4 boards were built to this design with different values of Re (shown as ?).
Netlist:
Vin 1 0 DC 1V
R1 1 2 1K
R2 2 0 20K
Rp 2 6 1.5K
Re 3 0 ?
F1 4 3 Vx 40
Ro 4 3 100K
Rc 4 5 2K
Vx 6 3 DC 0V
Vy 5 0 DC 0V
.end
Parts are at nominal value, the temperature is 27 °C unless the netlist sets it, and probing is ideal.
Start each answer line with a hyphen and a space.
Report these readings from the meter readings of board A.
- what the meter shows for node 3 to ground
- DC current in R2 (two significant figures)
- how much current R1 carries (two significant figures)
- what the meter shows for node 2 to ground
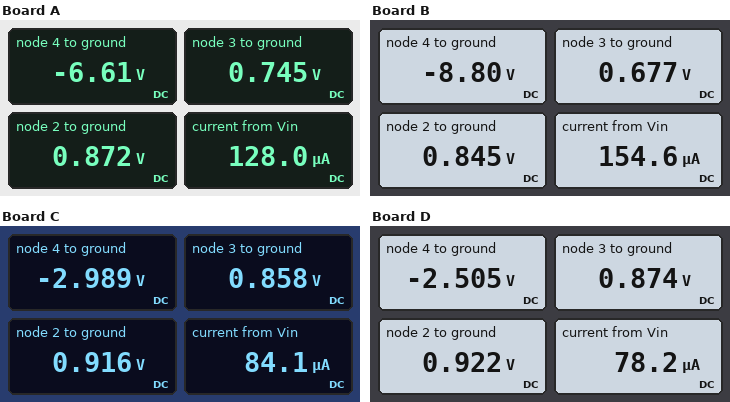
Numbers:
- 0.745 V
- 44 µA
- 130 µA
- 0.872 V
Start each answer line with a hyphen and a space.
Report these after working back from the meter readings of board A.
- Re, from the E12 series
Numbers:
- 220 Ω
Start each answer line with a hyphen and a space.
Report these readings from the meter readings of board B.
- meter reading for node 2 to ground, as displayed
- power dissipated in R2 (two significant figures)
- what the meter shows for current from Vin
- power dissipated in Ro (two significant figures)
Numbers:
- 0.845 V
- 36 µW
- 154.6 µA
- 900 µW
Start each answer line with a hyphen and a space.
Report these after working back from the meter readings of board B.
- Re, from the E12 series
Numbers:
- 150 Ω
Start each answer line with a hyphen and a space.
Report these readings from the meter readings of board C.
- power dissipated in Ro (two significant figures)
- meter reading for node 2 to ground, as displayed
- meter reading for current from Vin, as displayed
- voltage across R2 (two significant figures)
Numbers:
- 150 µW
- 0.916 V
- 84.1 µA
- 920 mV
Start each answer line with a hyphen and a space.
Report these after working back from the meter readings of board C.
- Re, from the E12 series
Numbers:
- 560 Ω
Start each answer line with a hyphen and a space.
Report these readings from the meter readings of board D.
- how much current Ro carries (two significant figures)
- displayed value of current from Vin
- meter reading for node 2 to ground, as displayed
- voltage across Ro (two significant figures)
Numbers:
- 34 µA
- 78.2 µA
- 0.922 V
- 3.4 V
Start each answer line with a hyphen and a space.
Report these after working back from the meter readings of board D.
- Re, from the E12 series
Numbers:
- 680 Ω
